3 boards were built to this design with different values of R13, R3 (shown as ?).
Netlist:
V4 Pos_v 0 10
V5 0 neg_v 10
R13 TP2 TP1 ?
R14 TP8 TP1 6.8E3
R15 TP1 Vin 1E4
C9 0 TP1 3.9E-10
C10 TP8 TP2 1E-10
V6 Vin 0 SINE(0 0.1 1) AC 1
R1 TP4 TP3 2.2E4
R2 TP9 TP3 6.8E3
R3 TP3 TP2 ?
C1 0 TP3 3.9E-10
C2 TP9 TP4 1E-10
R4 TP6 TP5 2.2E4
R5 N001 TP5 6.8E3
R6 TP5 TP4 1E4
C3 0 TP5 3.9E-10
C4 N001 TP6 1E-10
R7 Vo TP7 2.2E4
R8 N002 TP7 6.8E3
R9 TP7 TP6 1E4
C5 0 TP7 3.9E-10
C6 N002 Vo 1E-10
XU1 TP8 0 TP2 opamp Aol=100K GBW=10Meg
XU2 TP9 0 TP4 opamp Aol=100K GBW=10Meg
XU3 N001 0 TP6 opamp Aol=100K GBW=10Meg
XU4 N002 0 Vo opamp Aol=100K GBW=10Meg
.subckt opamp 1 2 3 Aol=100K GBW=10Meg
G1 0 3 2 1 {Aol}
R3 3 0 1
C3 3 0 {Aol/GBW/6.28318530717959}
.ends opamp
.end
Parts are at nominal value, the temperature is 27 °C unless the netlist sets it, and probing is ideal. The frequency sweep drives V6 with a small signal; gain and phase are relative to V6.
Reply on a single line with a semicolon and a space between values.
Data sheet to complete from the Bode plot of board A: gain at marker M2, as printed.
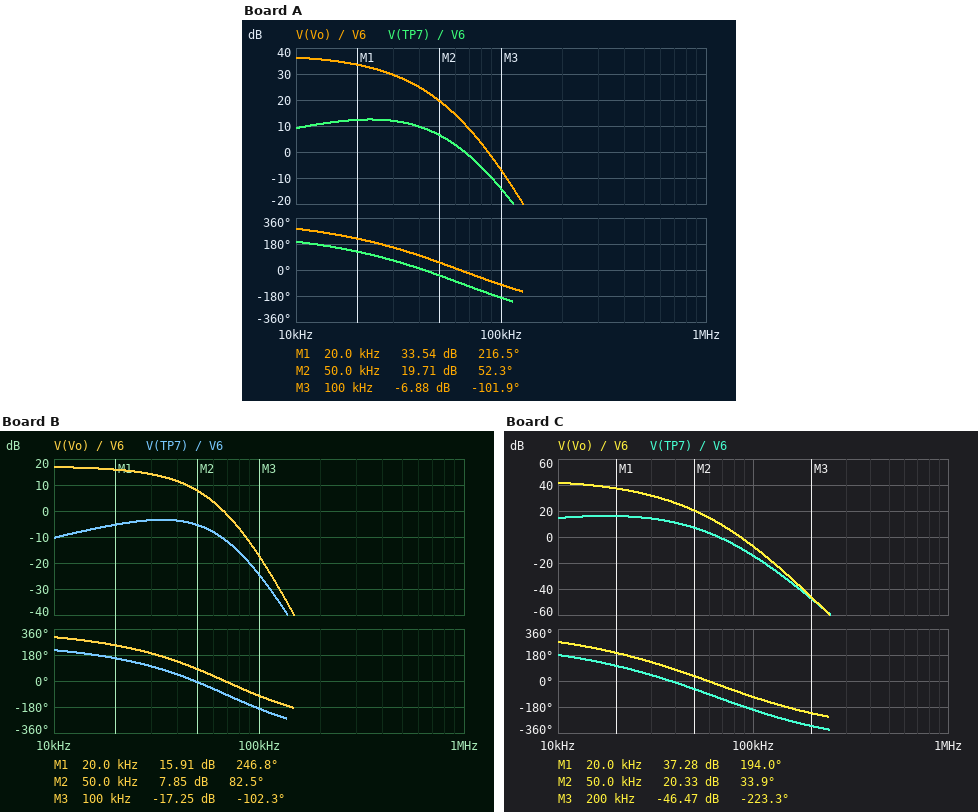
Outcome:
19.71 dB
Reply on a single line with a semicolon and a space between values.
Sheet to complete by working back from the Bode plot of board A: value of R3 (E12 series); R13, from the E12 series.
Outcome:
3.9 kΩ; 27 kΩ
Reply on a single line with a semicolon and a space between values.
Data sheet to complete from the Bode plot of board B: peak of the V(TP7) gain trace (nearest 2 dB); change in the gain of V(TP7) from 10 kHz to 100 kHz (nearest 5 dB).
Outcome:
-4 dB; -15 dB
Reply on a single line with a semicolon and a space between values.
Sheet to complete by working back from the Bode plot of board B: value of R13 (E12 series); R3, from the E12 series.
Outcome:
15 kΩ; 22 kΩ
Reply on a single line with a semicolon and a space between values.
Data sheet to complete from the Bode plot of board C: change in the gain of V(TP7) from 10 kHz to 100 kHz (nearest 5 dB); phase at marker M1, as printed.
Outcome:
-30 dB; 194.0 deg
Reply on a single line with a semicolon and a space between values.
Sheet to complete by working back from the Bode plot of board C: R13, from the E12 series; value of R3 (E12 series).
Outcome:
56 kΩ; 3.9 kΩ
